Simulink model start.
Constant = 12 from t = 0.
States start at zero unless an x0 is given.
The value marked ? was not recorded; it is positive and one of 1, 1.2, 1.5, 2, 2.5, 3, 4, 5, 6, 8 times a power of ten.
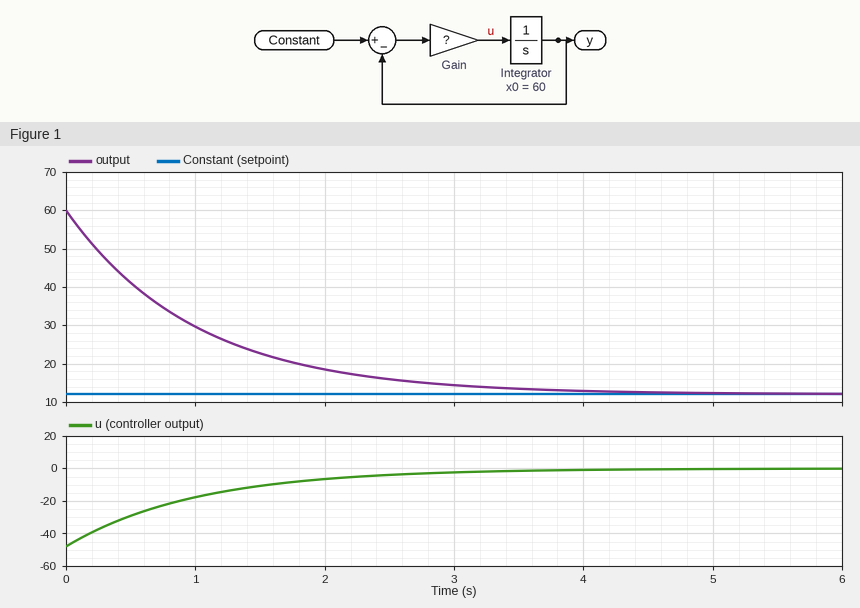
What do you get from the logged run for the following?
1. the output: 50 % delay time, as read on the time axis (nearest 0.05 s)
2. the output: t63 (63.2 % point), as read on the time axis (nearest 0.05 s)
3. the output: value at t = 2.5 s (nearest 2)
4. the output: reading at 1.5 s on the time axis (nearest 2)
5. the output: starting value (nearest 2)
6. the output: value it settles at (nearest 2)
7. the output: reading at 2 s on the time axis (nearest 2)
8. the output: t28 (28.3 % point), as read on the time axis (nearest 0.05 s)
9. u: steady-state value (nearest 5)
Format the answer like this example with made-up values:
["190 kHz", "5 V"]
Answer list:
["0.70 s", "1.00 s", "16", "22", "60", "12", "18", "0.35 s", "0"]
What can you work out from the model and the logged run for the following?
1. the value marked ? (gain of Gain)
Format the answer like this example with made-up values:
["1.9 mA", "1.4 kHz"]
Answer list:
["1"]
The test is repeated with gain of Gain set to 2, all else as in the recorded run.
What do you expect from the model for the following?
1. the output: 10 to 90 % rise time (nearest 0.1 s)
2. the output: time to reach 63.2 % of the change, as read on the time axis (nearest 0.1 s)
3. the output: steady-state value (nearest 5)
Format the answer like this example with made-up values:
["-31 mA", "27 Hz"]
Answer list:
["1.1 s", "0.5 s", "10"]
